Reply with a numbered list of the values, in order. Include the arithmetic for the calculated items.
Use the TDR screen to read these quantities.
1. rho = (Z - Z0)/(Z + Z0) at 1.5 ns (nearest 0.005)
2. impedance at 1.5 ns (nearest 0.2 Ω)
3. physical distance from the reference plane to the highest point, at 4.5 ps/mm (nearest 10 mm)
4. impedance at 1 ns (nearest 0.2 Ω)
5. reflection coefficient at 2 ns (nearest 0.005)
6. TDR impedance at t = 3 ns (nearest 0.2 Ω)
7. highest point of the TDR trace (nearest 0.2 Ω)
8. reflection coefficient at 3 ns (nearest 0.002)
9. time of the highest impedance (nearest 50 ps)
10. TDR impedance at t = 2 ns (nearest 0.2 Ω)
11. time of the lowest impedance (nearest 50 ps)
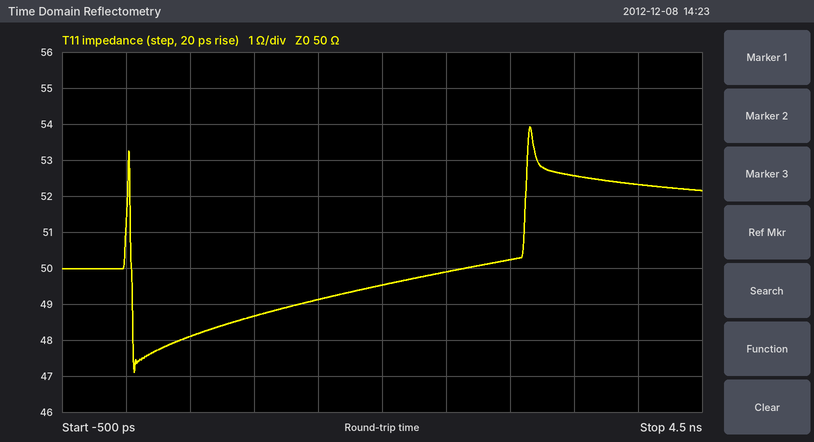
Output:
1. (49.2 − 50)/(49.2 + 50) ≈ -0.00806, so -0.010 to the nearest 0.005
2. 49.2 Ω
3. 3.15 ns / 2 / 4.5 ps/mm ≈ 350 mm
4. 48.6 Ω
5. (49.6 − 50)/(49.6 + 50) ≈ -0.00402, so -0.005 to the nearest 0.005
6. 50.2 Ω
7. 54.0 Ω
8. (50.2 − 50)/(50.2 + 50) ≈ +0.002
9. 3.15 ns
10. 49.6 Ω
11. 50 ps
